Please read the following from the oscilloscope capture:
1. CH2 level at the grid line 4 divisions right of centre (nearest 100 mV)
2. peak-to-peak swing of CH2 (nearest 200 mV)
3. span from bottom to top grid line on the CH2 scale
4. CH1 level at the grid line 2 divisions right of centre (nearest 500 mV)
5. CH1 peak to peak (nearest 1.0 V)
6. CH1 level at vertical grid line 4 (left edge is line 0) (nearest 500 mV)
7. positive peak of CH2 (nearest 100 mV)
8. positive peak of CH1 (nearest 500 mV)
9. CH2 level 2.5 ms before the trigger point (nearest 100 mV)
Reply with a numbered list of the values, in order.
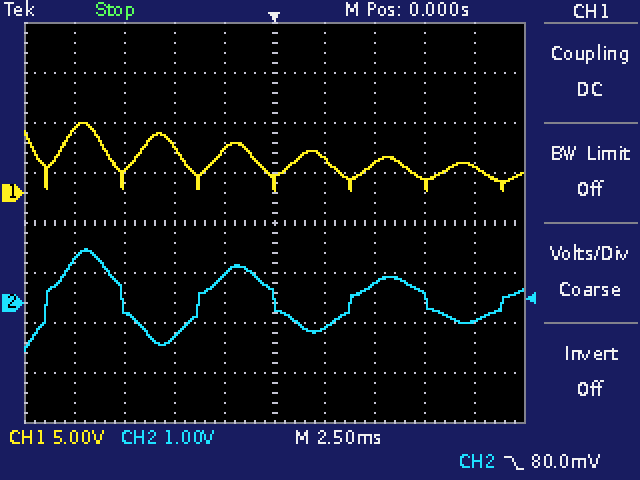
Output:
1. -400 mV
2. 2.0 V
3. 8 V
4. 3.0 V
5. 7.0 V
6. 4.5 V
7. 1.1 V
8. 7.0 V
9. 600 mV
